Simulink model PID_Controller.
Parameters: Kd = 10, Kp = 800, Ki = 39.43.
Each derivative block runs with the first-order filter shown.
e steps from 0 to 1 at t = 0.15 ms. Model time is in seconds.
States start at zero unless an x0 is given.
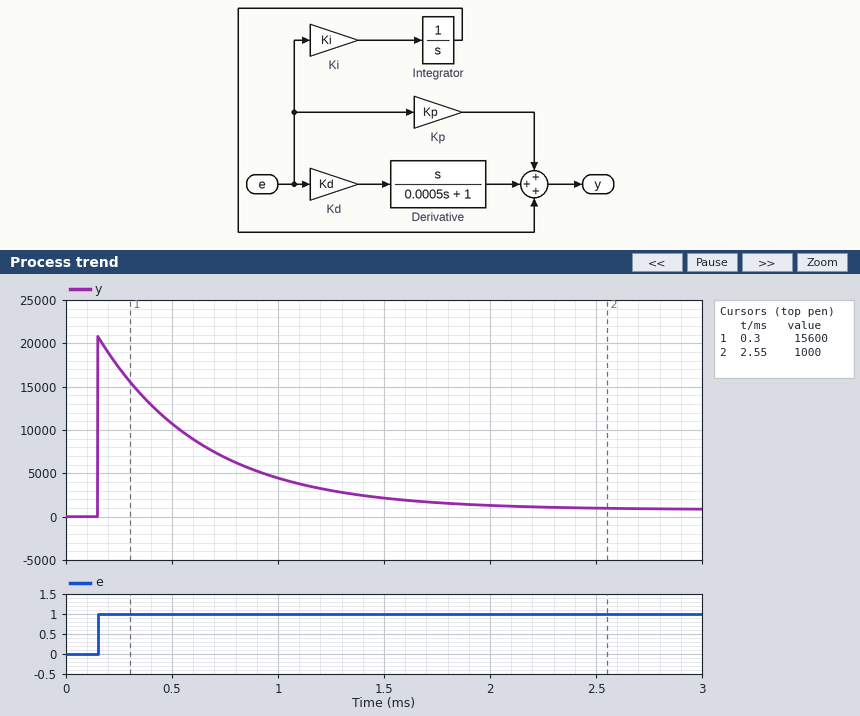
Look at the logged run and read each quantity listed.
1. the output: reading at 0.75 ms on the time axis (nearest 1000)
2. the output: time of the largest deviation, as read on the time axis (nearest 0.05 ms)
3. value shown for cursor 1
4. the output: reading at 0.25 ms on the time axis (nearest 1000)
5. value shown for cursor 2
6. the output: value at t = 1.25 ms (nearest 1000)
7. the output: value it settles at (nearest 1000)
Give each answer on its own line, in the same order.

7000
0.15 ms
15600
17000
1000
3000
1000
